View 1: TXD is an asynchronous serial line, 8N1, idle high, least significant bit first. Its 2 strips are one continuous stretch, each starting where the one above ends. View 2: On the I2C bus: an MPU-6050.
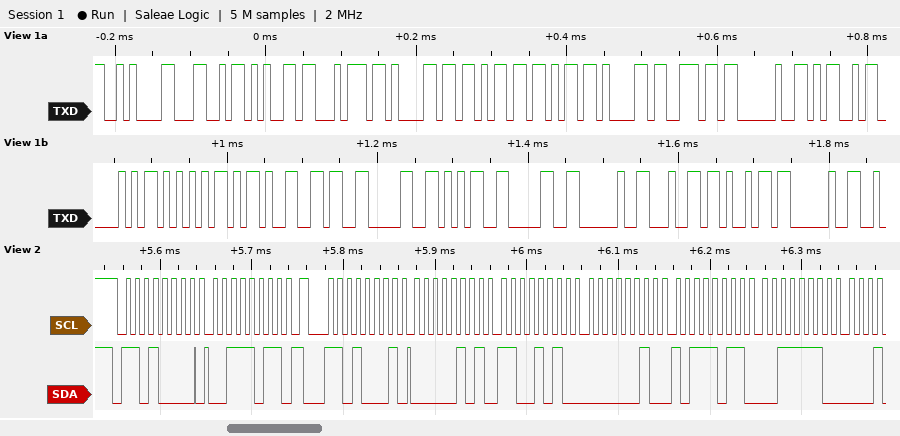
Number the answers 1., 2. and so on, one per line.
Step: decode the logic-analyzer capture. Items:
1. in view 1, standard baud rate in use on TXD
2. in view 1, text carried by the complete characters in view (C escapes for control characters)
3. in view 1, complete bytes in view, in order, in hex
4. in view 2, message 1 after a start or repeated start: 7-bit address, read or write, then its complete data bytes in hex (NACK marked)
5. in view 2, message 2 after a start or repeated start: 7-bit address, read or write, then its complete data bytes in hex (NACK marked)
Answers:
1. 115200 baud
2. "\nLetakkan MPU-6050 di "
3. 0x0A 0x4C 0x65 0x74 0x61 0x6B 0x6B 0x61 0x6E 0x20 0x4D 0x50 0x55 0x2D 0x36 0x30 0x35 0x30 0x20 0x64 0x69 0x20
4. 0x68 write: 3B
5. 0x68 read: 05 CA 02 BB 3E
